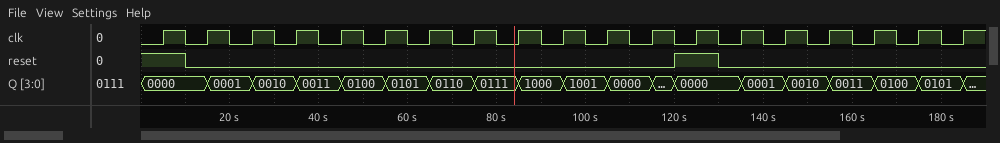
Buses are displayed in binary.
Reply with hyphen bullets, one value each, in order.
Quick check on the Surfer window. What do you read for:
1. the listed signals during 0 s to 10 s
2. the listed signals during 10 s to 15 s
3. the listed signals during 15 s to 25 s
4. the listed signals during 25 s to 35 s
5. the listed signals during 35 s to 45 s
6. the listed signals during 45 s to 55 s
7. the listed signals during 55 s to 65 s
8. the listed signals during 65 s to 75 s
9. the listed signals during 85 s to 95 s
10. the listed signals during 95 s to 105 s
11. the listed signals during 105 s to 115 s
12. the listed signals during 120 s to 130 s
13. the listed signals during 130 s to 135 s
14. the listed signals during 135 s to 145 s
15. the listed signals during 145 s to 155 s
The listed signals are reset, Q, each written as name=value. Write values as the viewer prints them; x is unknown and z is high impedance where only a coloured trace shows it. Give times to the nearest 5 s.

- reset=1, Q=0000
- reset=0, Q=0000
- reset=0, Q=0001
- reset=0, Q=0010
- reset=0, Q=0011
- reset=0, Q=0100
- reset=0, Q=0101
- reset=0, Q=0110
- reset=0, Q=1000
- reset=0, Q=1001
- reset=0, Q=0000
- reset=1, Q=0000
- reset=0, Q=0000
- reset=0, Q=0001
- reset=0, Q=0010
